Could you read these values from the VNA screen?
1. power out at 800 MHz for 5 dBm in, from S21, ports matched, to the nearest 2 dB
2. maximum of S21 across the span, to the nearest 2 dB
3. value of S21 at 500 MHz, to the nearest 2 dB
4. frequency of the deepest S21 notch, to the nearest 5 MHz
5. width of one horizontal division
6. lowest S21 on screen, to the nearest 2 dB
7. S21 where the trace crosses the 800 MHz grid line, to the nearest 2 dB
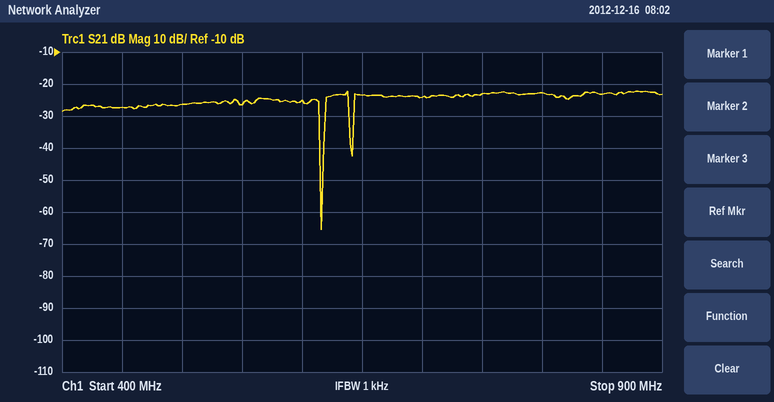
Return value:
-18 dBm
-22 dB
-26 dB
615 MHz
50 MHz
-66 dB
-22 dB
